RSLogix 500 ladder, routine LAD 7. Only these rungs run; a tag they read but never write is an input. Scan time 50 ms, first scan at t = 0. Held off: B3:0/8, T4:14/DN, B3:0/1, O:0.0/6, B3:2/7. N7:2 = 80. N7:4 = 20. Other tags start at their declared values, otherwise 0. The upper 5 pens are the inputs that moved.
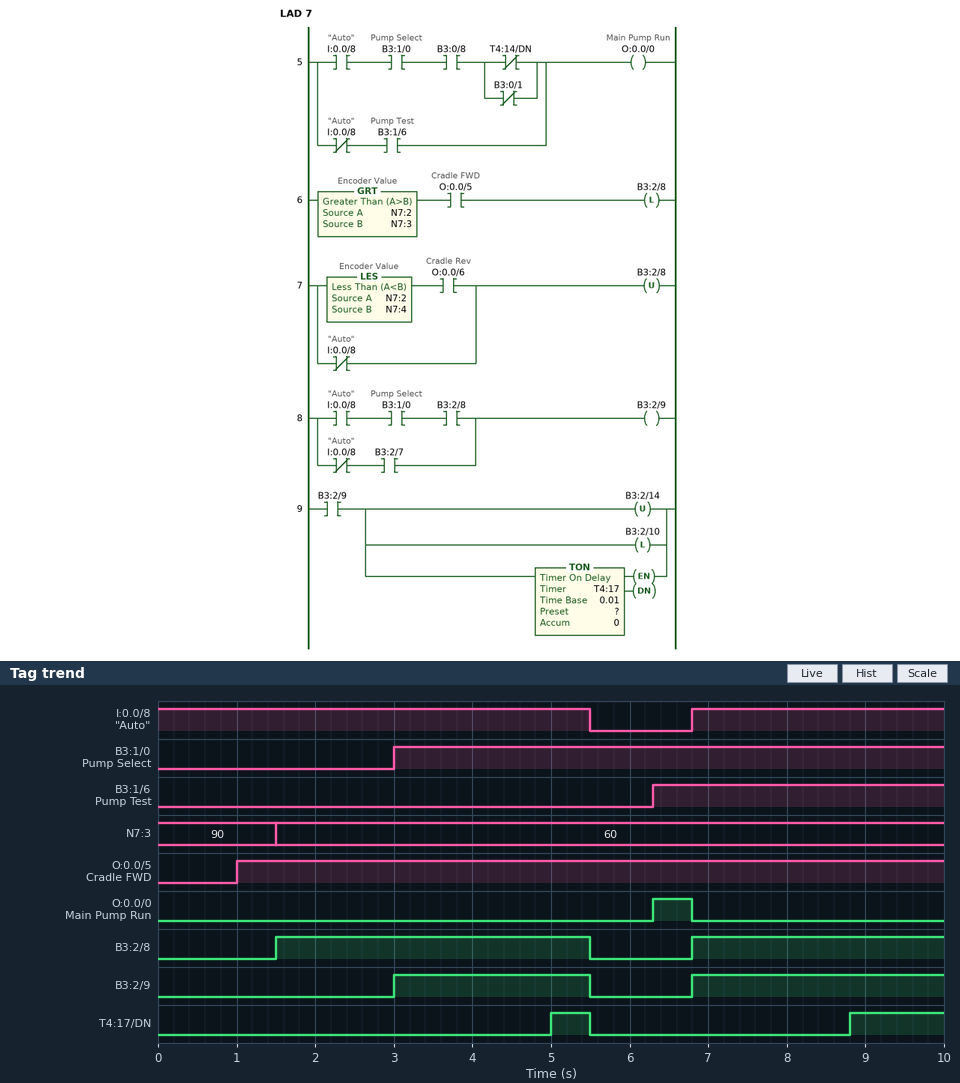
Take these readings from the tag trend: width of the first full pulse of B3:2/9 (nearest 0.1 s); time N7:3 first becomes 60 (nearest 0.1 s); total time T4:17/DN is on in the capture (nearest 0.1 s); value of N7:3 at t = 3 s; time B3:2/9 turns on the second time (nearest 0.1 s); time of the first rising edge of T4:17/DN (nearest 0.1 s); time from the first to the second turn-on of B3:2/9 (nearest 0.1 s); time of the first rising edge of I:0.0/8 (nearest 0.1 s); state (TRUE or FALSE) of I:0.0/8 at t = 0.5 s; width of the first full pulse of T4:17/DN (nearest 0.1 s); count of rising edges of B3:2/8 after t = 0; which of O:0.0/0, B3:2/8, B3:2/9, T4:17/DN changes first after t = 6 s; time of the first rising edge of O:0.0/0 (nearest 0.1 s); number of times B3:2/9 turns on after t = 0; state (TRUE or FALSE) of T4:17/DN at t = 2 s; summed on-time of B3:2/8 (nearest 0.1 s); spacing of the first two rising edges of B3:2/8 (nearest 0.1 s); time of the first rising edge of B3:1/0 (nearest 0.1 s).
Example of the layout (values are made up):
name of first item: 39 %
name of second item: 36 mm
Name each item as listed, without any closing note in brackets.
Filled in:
width of the first full pulse of B3:2/9: 2.5 s
time N7:3 first becomes 60: 1.5 s
total time T4:17/DN is on in the capture: 1.7 s
value of N7:3 at t = 3 s: 60
time B3:2/9 turns on the second time: 6.8 s
time of the first rising edge of T4:17/DN: 5.0 s
time from the first to the second turn-on of B3:2/9: 3.8 s
time of the first rising edge of I:0.0/8: 6.8 s
state (TRUE or FALSE) of I:0.0/8 at t = 0.5 s: TRUE
width of the first full pulse of T4:17/DN: 0.5 s
count of rising edges of B3:2/8 after t = 0: 2
which of O:0.0/0, B3:2/8, B3:2/9, T4:17/DN changes first after t = 6 s: O:0.0/0
time of the first rising edge of O:0.0/0: 6.3 s
number of times B3:2/9 turns on after t = 0: 2
state (TRUE or FALSE) of T4:17/DN at t = 2 s: FALSE
summed on-time of B3:2/8: 7.2 s
spacing of the first two rising edges of B3:2/8: 5.3 s
time of the first rising edge of B3:1/0: 3.0 s
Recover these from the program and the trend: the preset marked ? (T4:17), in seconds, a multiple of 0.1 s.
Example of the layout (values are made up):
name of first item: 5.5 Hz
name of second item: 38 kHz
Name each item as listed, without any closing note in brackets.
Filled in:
the preset marked ? (T4:17), in seconds, a multiple of 0.1 s: 2.0 s
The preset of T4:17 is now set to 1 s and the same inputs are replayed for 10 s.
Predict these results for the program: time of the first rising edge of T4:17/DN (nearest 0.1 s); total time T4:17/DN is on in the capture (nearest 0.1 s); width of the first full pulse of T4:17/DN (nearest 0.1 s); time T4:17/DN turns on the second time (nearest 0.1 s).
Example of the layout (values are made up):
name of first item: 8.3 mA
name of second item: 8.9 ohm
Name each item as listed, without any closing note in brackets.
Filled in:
time of the first rising edge of T4:17/DN: 4.0 s
total time T4:17/DN is on in the capture: 3.7 s
width of the first full pulse of T4:17/DN: 1.5 s
time T4:17/DN turns on the second time: 7.8 s
